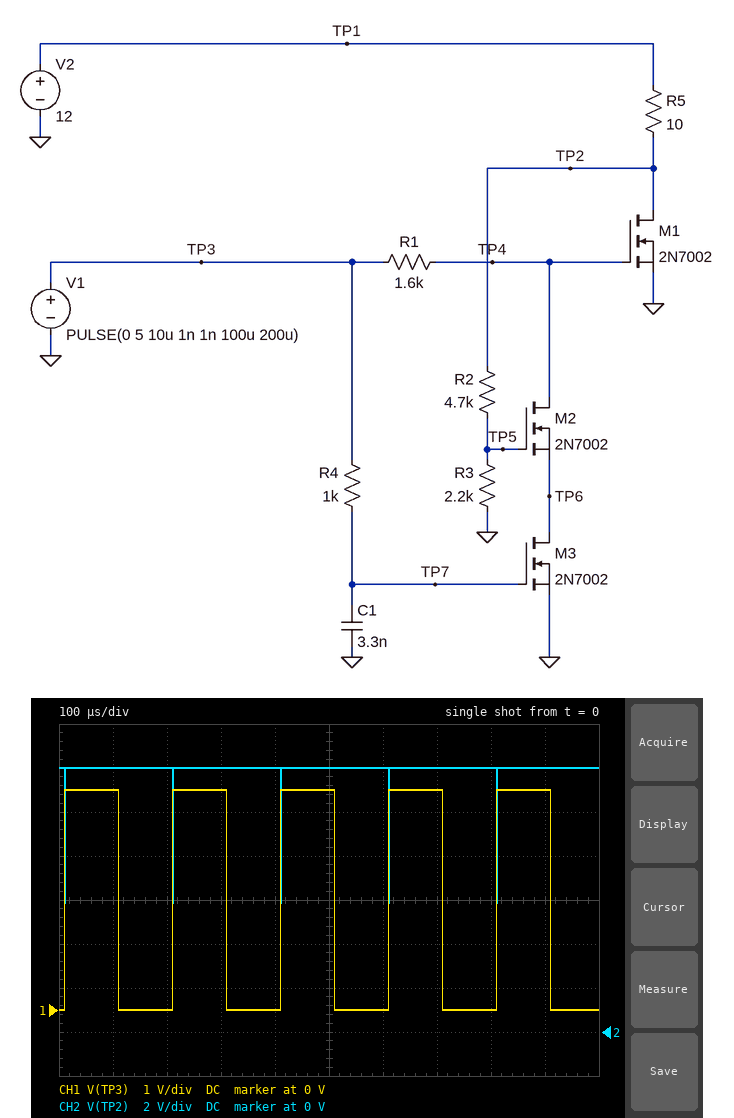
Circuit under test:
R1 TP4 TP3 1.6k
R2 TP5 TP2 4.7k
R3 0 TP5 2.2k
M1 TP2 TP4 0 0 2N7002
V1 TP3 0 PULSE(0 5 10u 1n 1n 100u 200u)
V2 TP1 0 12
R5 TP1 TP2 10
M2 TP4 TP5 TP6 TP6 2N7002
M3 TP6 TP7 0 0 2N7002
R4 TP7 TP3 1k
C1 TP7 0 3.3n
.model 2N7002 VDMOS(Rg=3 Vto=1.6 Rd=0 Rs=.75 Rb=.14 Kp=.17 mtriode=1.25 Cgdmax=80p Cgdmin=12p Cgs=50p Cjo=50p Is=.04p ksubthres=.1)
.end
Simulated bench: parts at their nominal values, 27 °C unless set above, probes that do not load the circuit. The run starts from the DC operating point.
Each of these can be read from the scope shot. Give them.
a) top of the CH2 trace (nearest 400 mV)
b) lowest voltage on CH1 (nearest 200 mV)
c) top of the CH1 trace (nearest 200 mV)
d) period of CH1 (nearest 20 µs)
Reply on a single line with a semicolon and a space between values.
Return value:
12.0 V; 0 V; 5.0 V; 200 µs
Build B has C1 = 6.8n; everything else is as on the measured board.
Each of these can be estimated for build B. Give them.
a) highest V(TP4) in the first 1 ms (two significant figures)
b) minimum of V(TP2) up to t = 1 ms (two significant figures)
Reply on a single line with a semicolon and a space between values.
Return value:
5.0 V; 5.1 V
